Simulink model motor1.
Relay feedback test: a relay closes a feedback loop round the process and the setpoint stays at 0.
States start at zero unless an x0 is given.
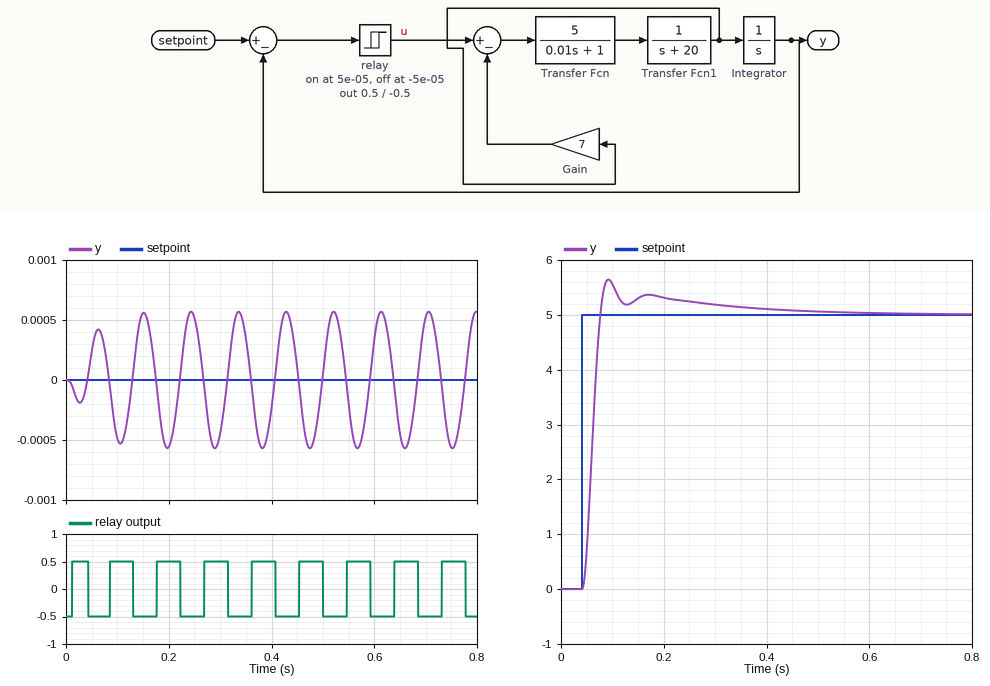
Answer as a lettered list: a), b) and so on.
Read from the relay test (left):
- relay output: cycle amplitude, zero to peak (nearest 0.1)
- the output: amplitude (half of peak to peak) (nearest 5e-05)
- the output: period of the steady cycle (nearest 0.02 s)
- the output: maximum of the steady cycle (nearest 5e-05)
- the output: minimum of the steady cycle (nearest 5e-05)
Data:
a) 0.5
b) 0.00055
c) 0.10 s
d) 0.00055
e) -0.00055
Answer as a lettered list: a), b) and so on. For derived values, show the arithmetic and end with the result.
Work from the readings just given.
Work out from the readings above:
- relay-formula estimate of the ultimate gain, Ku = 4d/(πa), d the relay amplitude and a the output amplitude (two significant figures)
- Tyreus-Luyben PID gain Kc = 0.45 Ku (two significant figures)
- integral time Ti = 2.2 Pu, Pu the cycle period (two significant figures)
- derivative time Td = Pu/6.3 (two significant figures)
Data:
a) 4 × 0.5 / (π × 0.00055) = 1200
b) 0.45 × 1200 = 540
c) 2.2 × 0.1 = 0.22 s
d) 0.1 / 6.3 = 0.016 s
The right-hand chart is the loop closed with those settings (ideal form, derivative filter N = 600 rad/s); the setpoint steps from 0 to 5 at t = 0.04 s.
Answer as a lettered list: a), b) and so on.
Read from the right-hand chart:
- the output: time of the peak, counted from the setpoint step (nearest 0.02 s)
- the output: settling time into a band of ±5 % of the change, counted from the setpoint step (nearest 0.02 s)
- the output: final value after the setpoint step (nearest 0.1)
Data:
a) 0.06 s
b) 0.20 s
c) 5.0
